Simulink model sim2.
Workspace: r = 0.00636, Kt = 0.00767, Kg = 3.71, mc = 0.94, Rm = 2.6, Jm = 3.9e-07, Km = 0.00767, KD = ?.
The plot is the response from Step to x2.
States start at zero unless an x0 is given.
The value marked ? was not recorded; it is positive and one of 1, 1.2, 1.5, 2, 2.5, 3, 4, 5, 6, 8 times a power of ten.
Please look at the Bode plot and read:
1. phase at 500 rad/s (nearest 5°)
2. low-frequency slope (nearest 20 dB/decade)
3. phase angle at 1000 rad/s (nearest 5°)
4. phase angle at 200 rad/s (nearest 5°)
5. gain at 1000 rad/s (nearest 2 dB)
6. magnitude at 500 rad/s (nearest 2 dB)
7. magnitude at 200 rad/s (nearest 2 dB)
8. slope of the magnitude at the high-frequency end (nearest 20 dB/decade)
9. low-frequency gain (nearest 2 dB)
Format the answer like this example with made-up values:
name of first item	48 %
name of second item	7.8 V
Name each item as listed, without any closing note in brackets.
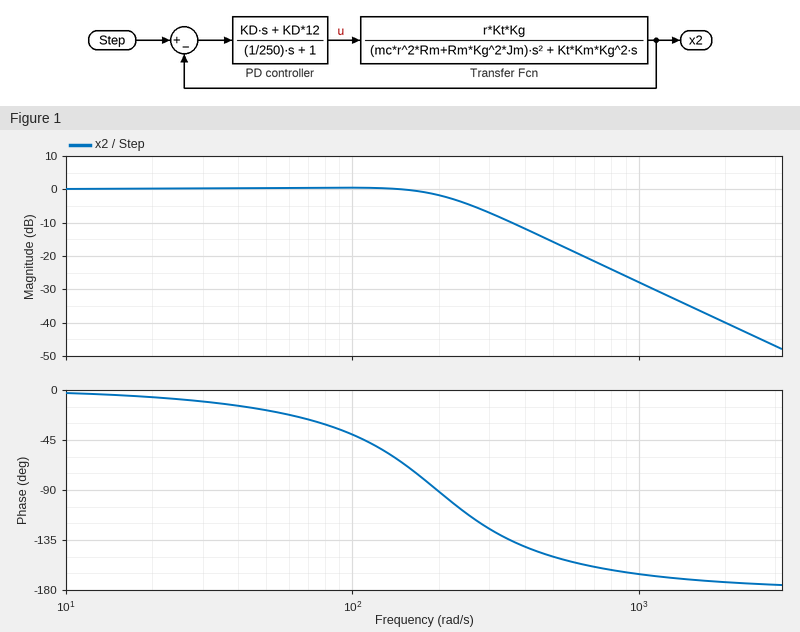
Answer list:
phase at 500 rad/s	-150°
low-frequency slope	0 dB/decade
phase angle at 1000 rad/s	-165°
phase angle at 200 rad/s	-90°
gain at 1000 rad/s	-28 dB
magnitude at 500 rad/s	-16 dB
magnitude at 200 rad/s	-2 dB
slope of the magnitude at the high-frequency end	-40 dB/decade
low-frequency gain	0 dB
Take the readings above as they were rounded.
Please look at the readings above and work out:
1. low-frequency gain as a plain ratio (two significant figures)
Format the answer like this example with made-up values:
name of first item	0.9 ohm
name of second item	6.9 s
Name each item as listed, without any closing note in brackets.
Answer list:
low-frequency gain as a plain ratio	1.0
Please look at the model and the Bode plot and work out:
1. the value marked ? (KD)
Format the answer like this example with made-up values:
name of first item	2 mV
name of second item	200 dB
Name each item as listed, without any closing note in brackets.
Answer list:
the value marked ?	100
